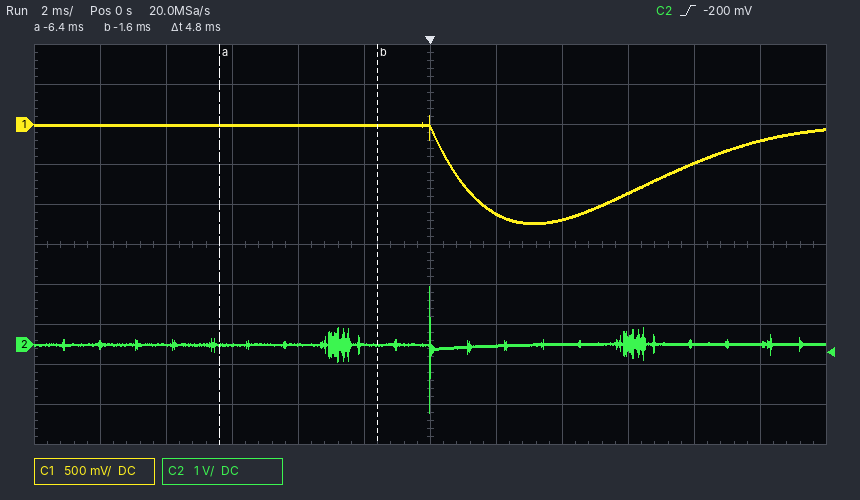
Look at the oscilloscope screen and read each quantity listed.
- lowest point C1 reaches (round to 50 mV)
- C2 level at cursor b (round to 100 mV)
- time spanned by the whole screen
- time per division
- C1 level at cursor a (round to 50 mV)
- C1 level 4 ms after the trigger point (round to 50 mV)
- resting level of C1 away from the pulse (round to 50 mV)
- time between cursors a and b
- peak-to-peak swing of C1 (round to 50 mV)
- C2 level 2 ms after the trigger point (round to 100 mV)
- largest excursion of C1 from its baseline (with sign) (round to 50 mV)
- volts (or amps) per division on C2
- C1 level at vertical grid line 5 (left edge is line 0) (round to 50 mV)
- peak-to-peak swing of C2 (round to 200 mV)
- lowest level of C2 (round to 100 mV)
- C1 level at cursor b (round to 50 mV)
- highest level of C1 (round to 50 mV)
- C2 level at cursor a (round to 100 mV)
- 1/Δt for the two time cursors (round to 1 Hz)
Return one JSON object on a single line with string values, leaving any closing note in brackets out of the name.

{"lowest point C1 reaches": "-1.25 V", "C2 level at cursor b": "0.0 V", "time spanned by the whole screen": "24 ms", "time per division": "2 ms", "C1 level at cursor a": "0 mV", "C1 level 4 ms after the trigger point": "-1.20 V", "resting level of C1 away from the pulse": "0 mV", "time between cursors a and b": "4.8 ms", "peak-to-peak swing of C1": "1.35 V", "C2 level 2 ms after the trigger point": "0.0 V", "largest excursion of C1 from its baseline (with sign)": "-1.25 V", "volts (or amps) per division on C2": "1 V", "C1 level at vertical grid line 5 (left edge is line 0)": "0 mV", "peak-to-peak swing of C2": "3.2 V", "lowest level of C2": "-1.7 V", "C1 level at cursor b": "0 mV", "highest level of C1": "100 mV", "C2 level at cursor a": "0.0 V", "1/Δt for the two time cursors": "208 Hz"}
